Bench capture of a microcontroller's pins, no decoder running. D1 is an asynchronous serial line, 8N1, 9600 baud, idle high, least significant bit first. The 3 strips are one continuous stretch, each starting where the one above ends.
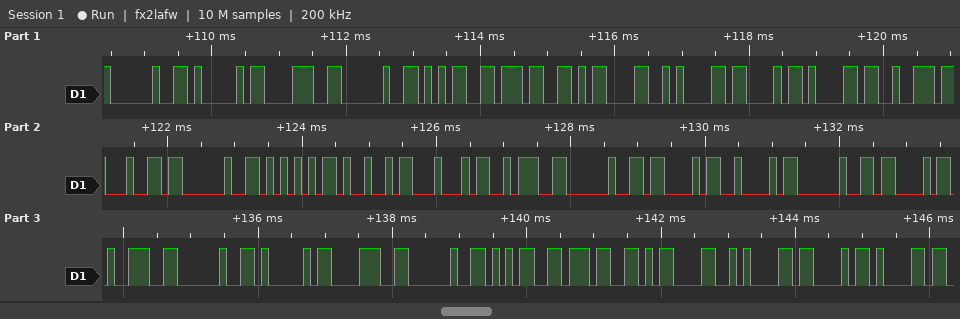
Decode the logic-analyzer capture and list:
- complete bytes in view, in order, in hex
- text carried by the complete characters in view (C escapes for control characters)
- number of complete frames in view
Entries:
20 41 38 20 35 37 0D 0A 43 61 72 64 20 55 49 44 3A 20 43 42 20 43 39 20 41 38 20 35 37 0D 0A 43 61
" A8 57\r\nCard UID: CB C9 A8 57\r\nCa"
33
